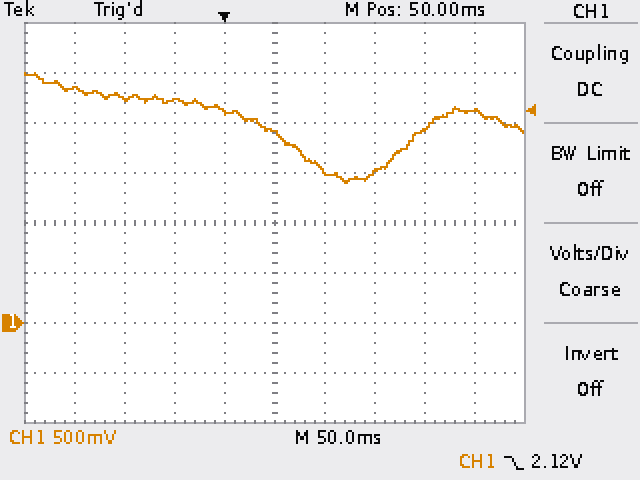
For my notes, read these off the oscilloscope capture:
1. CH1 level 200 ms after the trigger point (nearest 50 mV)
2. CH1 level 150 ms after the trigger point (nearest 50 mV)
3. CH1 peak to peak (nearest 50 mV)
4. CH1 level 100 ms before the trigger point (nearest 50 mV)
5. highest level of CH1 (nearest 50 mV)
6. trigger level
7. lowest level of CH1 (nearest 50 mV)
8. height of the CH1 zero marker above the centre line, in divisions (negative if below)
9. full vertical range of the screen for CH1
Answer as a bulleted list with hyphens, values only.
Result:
- 1.95 V
- 1.50 V
- 1.10 V
- 2.25 V
- 2.50 V
- 2.12 V
- 1.40 V
- -2.0 div
- 4 V
